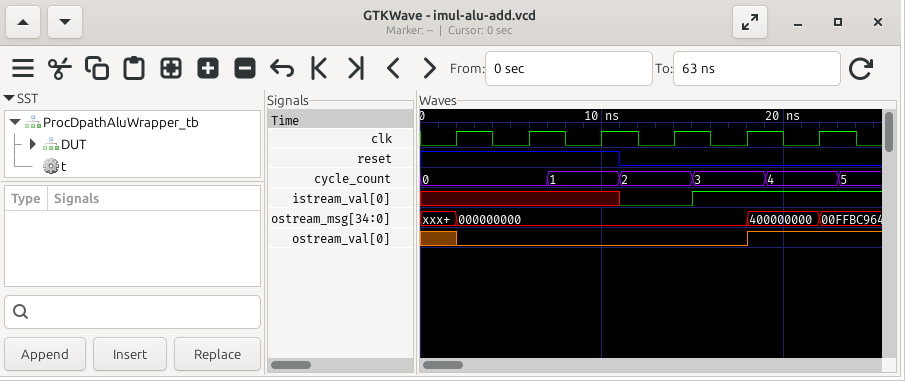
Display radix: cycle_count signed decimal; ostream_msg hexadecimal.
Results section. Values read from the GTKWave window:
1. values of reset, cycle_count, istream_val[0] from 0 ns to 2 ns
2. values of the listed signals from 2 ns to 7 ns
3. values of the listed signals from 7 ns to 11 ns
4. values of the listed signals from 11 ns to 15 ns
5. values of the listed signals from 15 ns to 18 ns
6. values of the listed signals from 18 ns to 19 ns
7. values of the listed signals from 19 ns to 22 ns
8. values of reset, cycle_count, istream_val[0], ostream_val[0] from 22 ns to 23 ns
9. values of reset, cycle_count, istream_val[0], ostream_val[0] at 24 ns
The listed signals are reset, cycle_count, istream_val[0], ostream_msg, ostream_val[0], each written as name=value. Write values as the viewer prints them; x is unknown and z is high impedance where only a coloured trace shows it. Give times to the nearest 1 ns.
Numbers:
reset=1, cycle_count=0, istream_val[0]=x
reset=1, cycle_count=0, istream_val[0]=x, ostream_msg=000000000, ostream_val[0]=0
reset=1, cycle_count=1, istream_val[0]=x, ostream_msg=000000000, ostream_val[0]=0
reset=0, cycle_count=2, istream_val[0]=0, ostream_msg=000000000, ostream_val[0]=0
reset=0, cycle_count=3, istream_val[0]=1, ostream_msg=000000000, ostream_val[0]=0
reset=0, cycle_count=3, istream_val[0]=1, ostream_msg=400000000, ostream_val[0]=1
reset=0, cycle_count=4, istream_val[0]=1, ostream_msg=400000000, ostream_val[0]=1
reset=0, cycle_count=4, istream_val[0]=1, ostream_val[0]=1
reset=0, cycle_count=5, istream_val[0]=1, ostream_val[0]=1
